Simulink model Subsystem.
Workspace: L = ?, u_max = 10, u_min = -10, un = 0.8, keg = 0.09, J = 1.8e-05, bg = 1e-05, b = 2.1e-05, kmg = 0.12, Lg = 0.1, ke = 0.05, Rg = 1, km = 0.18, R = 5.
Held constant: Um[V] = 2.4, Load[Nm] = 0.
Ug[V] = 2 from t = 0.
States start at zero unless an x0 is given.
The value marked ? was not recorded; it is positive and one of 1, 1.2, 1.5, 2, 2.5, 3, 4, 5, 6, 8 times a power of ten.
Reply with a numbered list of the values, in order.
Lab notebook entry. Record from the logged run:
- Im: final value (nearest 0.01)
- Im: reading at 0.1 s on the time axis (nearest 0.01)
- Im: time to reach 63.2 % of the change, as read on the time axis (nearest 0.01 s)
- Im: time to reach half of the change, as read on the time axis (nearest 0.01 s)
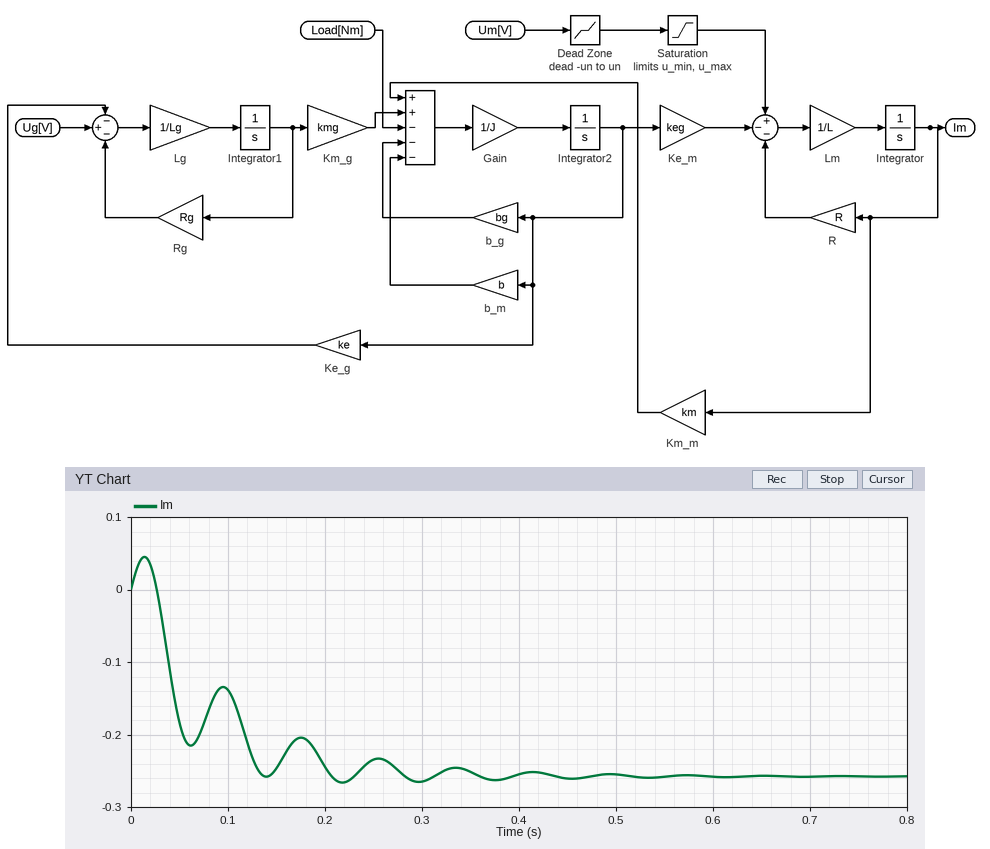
1. -0.26
2. -0.14
3. 0.05 s
4. 0.04 s
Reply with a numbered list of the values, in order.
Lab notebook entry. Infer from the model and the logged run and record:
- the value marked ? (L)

1. 0.3
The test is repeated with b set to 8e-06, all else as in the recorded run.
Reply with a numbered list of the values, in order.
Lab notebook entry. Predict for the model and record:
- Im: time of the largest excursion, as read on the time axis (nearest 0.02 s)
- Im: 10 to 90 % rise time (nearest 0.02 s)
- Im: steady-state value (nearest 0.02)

1. 0.22 s
2. 0.10 s
3. -0.26
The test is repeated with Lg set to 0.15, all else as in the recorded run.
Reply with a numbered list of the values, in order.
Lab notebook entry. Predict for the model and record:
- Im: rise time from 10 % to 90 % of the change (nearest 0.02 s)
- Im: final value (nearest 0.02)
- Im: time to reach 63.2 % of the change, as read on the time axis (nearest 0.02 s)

1. 0.10 s
2. -0.26
3. 0.06 s
